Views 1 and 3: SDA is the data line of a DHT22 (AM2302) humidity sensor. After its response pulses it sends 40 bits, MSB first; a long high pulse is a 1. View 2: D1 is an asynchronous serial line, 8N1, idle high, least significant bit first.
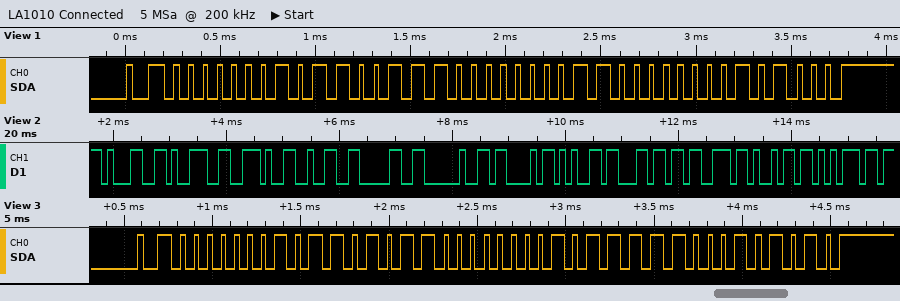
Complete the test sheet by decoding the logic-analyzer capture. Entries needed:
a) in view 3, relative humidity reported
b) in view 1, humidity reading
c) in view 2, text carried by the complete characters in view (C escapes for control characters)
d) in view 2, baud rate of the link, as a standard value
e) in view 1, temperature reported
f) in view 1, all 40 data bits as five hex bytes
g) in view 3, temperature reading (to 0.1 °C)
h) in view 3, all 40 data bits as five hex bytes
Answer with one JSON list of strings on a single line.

["36.3 %", "35.9 %", "\"19.20 Celsiu\"", "9600 baud", "19.2 °C", "01 67 00 C0 28", "19.0 °C", "01 6B 00 BE 2A"]
